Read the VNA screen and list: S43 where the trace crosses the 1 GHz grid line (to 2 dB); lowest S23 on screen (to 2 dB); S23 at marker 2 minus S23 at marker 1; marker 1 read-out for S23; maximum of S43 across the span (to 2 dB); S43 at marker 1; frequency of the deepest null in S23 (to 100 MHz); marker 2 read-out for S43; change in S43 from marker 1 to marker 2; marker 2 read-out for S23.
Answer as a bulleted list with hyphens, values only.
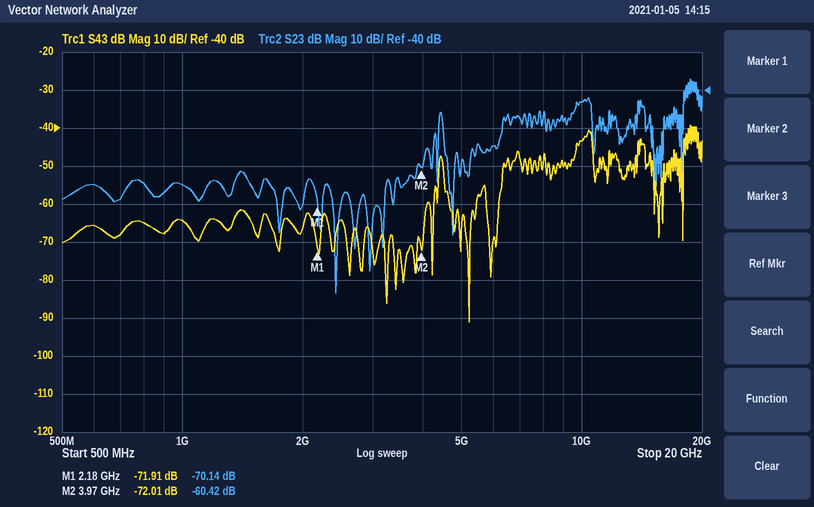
- -64 dB
- -94 dB
- 9.72 dB
- -70.14 dB
- -40 dB
- -71.91 dB
- 2.4 GHz
- -72.01 dB
- -0.10 dB
- -60.42 dB
